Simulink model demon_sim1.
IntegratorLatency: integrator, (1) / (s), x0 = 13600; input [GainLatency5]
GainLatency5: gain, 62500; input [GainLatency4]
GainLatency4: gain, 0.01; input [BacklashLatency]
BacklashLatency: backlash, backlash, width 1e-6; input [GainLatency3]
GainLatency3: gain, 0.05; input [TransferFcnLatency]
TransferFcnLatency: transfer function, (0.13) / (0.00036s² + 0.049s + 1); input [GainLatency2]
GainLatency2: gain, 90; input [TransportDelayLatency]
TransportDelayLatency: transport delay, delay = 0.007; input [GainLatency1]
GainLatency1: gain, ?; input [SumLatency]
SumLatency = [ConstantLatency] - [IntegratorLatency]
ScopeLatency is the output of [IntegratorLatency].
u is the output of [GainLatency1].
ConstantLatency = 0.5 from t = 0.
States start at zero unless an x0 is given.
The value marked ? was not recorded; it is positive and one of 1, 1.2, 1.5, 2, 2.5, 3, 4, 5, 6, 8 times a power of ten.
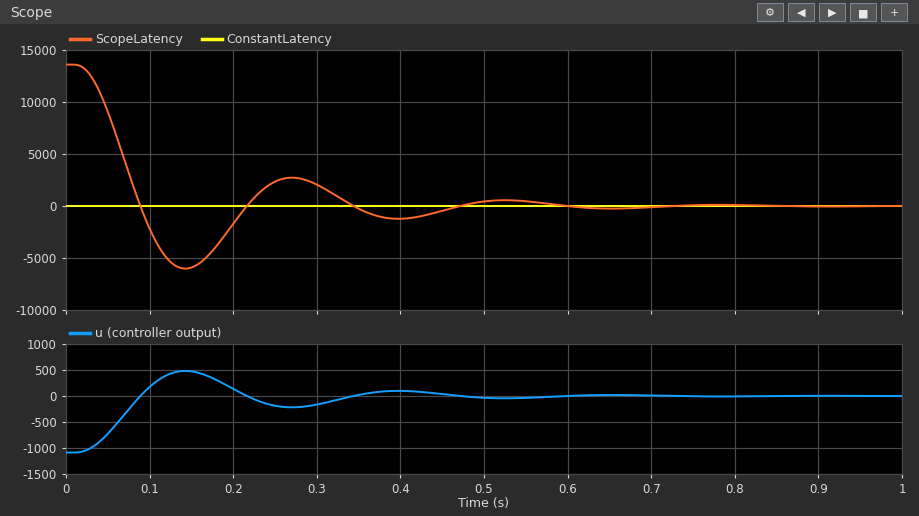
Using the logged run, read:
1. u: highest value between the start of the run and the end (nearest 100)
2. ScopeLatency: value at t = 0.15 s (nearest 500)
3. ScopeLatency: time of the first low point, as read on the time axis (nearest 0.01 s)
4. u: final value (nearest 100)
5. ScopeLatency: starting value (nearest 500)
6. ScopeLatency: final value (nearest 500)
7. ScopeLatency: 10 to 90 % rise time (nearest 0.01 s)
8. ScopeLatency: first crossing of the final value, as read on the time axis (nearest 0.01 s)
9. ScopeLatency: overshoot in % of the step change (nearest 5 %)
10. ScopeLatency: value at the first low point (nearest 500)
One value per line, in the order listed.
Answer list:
500
-6000
0.14 s
0
13500
0
0.05 s
0.09 s
45 %
-6000
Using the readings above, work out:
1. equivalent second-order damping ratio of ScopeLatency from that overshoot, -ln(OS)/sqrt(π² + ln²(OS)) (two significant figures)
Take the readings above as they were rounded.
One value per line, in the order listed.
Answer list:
0.25
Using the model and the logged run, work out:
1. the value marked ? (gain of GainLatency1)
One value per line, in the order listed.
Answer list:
0.08
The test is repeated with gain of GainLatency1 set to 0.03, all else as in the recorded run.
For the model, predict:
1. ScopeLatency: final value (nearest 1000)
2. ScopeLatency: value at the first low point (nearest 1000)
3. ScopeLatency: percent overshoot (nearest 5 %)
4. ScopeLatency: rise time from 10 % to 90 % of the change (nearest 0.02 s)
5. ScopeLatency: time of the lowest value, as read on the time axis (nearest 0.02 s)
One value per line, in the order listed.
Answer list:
0
-1000
10 %
0.12 s
0.26 s
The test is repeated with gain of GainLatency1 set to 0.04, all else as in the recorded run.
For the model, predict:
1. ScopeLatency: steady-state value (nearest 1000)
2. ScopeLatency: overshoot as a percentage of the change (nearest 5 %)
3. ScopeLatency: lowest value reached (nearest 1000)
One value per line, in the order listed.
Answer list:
0
15 %
-2000
